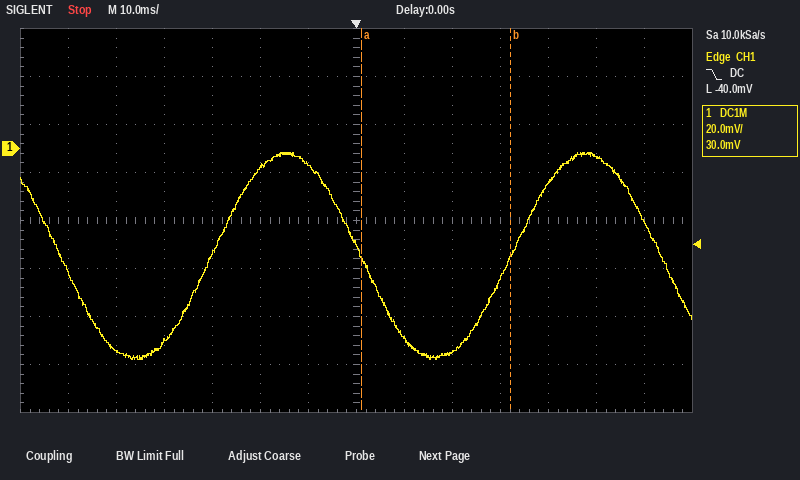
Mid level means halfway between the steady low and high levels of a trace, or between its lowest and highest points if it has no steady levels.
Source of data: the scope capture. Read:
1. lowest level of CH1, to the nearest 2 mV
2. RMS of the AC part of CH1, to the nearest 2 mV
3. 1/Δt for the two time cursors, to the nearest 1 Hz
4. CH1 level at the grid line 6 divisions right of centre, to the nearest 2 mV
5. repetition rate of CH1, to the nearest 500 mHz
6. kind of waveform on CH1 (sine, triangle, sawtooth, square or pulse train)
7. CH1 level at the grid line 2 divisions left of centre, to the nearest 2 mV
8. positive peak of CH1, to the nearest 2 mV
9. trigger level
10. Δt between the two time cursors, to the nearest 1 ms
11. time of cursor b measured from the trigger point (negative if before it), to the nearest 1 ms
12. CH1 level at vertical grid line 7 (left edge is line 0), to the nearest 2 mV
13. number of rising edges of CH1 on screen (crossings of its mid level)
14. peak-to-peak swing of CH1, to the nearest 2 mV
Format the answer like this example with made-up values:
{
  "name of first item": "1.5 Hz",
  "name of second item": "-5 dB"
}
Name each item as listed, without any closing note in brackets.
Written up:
{
  "lowest level of CH1, to the nearest 2 mV": "-88 mV",
  "RMS of the AC part of CH1, to the nearest 2 mV": "30 mV",
  "1/Δt for the two time cursors, to the nearest 1 Hz": "32 Hz",
  "CH1 level at the grid line 6 divisions right of centre, to the nearest 2 mV": "-30 mV",
  "repetition rate of CH1, to the nearest 500 mHz": "16.0 Hz",
  "kind of waveform on CH1": "sine",
  "CH1 level at the grid line 2 divisions left of centre, to the nearest 2 mV": "-8 mV",
  "positive peak of CH1, to the nearest 2 mV": "-2 mV",
  "trigger level": "-40.0 mV",
  "Δt between the two time cursors, to the nearest 1 ms": "31 ms",
  "time of cursor b measured from the trigger point (negative if before it), to the nearest 1 ms": "+32 ms",
  "CH1 level at vertical grid line 7 (left edge is line 0), to the nearest 2 mV": "-40 mV",
  "number of rising edges of CH1 on screen": "2",
  "peak-to-peak swing of CH1, to the nearest 2 mV": "86 mV"
}
